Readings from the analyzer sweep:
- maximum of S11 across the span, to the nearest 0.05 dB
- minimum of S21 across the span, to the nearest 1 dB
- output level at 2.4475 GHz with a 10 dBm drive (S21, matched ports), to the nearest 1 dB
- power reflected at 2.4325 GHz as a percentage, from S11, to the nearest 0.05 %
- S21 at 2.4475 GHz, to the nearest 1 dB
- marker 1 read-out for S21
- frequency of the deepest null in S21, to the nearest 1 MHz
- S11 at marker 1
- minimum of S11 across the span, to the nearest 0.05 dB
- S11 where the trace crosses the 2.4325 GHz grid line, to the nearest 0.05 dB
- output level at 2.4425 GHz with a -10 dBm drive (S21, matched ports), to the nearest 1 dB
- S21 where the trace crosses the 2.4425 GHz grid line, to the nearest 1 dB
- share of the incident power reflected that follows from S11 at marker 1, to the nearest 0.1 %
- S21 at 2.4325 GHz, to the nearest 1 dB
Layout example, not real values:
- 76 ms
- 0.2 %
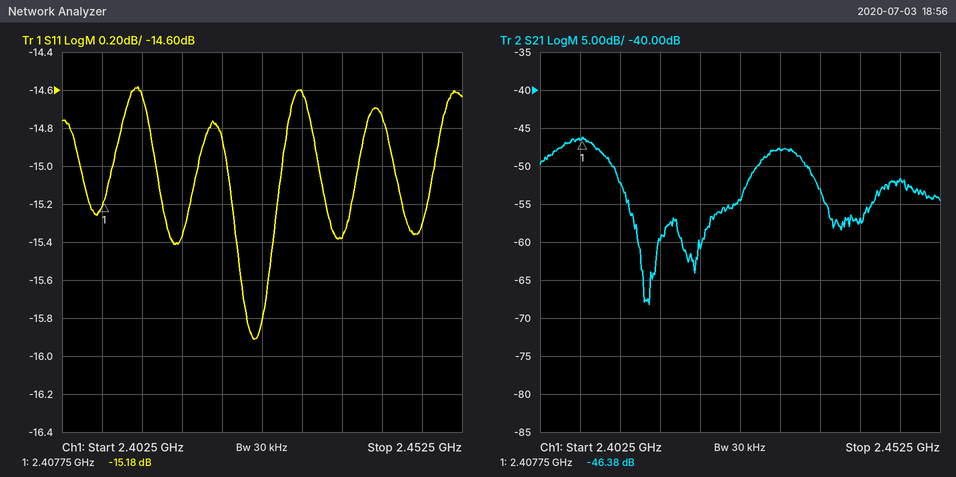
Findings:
- -14.60 dB
- -68 dB
- -42 dBm
- 3.45 %
- -52 dB
- -46.38 dB
- 2.416 GHz
- -15.18 dB
- -15.90 dB
- -14.60 dB
- -67 dBm
- -57 dB
- 3.0 %
- -48 dB
